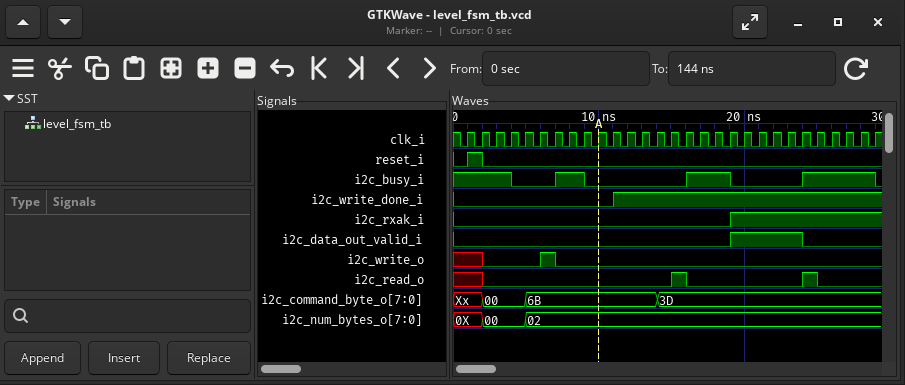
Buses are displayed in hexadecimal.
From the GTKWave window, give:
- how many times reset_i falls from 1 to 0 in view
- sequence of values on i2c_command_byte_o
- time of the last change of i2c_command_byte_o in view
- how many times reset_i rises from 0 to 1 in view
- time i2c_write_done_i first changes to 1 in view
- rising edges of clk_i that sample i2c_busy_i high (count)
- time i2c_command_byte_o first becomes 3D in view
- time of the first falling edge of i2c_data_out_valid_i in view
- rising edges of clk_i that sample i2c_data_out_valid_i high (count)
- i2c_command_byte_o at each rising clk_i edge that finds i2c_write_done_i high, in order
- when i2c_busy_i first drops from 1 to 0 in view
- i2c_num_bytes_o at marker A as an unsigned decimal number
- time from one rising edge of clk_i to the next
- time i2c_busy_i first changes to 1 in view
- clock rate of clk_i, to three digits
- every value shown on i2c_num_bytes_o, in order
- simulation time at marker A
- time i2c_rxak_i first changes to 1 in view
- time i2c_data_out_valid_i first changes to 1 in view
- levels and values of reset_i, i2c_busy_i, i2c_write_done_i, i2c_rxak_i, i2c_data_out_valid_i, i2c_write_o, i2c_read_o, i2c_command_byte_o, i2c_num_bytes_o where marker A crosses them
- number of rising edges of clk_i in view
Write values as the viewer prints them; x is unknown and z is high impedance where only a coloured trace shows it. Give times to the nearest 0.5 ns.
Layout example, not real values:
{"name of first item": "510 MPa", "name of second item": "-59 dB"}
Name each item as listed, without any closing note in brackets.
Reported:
{"how many times reset_i falls from 1 to 0 in view": "1", "sequence of values on i2c_command_byte_o": "Xx, 00, 6B, 3D", "time of the last change of i2c_command_byte_o in view": "14 ns", "how many times reset_i rises from 0 to 1 in view": "1", "time i2c_write_done_i first changes to 1 in view": "11 ns", "rising edges of clk_i that sample i2c_busy_i high": "14", "time i2c_command_byte_o first becomes 3D in view": "14 ns", "time of the first falling edge of i2c_data_out_valid_i in view": "24 ns", "rising edges of clk_i that sample i2c_data_out_valid_i high": "5", "i2c_command_byte_o at each rising clk_i edge that finds i2c_write_done_i high, in order": "6B, 6B, 6B, 3D, 3D, 3D, 3D, 3D, 3D, 3D, 3D, 3D, 3D, 3D, 3D, 3D, 3D, 3D", "when i2c_busy_i first drops from 1 to 0 in view": "4 ns", "i2c_num_bytes_o at marker A as an unsigned decimal number": "2", "time from one rising edge of clk_i to the next": "1 ns", "time i2c_busy_i first changes to 1 in view": "7 ns", "clock rate of clk_i, to three digits": "1.00 GHz", "every value shown on i2c_num_bytes_o, in order": "0X, 00, 02", "simulation time at marker A": "10 ns", "time i2c_rxak_i first changes to 1 in view": "19 ns", "time i2c_data_out_valid_i first changes to 1 in view": "19 ns", "levels and values of reset_i, i2c_busy_i, i2c_write_done_i, i2c_rxak_i, i2c_data_out_valid_i, i2c_write_o, i2c_read_o, i2c_command_byte_o, i2c_num_bytes_o where marker A crosses them": "reset_i=0, i2c_busy_i=0, i2c_write_done_i=0, i2c_rxak_i=0, i2c_data_out_valid_i=0, i2c_write_o=0, i2c_read_o=0, i2c_command_byte_o=6B, i2c_num_bytes_o=02", "number of rising edges of clk_i in view": "29"}
